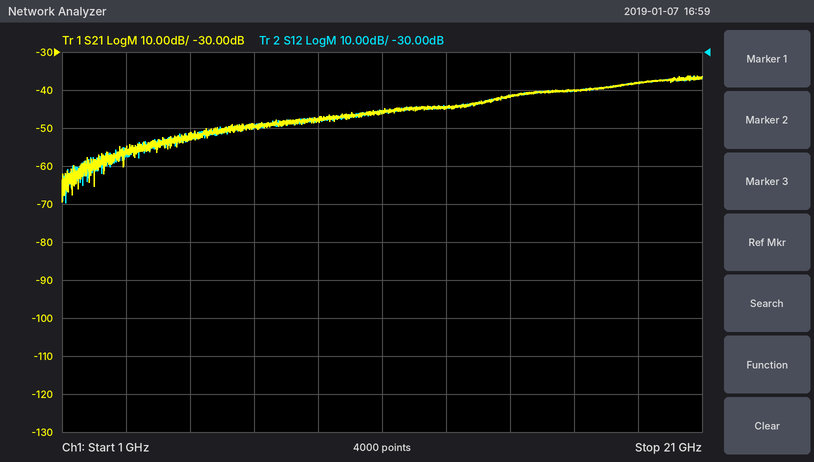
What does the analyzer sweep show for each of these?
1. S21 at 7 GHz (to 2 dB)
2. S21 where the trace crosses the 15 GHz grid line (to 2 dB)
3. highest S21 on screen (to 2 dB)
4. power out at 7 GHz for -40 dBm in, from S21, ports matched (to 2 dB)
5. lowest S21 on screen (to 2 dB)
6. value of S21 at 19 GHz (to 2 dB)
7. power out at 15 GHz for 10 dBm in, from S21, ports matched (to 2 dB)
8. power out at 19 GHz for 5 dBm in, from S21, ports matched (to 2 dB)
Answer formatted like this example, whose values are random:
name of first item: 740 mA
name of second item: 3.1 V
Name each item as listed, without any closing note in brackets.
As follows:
S21 at 7 GHz: -50 dB
S21 where the trace crosses the 15 GHz grid line: -42 dB
highest S21 on screen: -36 dB
power out at 7 GHz for -40 dBm in, from S21, ports matched: -90 dBm
lowest S21 on screen: -70 dB
value of S21 at 19 GHz: -38 dB
power out at 15 GHz for 10 dBm in, from S21, ports matched: -32 dBm
power out at 19 GHz for 5 dBm in, from S21, ports matched: -34 dBm
